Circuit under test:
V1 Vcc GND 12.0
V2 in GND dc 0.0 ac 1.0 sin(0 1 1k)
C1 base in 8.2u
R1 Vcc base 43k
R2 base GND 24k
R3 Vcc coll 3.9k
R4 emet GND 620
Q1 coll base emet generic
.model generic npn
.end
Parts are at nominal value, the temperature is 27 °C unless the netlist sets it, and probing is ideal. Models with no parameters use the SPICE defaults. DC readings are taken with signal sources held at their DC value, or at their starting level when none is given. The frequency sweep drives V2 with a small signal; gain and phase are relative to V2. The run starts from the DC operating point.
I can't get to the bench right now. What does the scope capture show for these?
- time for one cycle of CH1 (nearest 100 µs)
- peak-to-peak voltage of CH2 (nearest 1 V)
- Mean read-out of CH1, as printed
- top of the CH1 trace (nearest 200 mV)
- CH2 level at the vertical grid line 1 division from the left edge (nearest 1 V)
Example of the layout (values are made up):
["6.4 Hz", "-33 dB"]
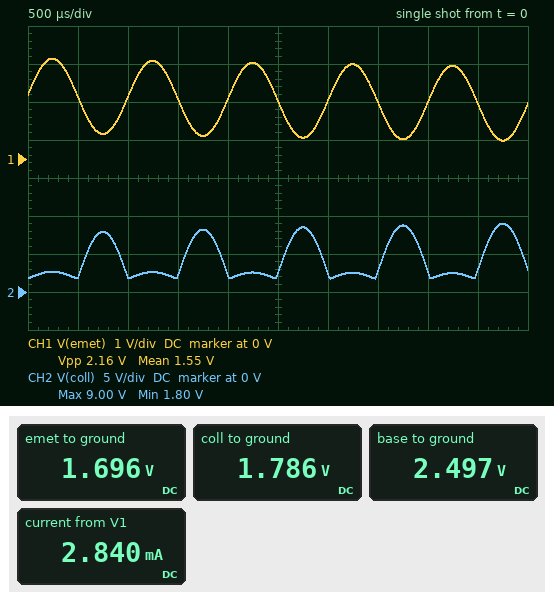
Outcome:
["1.0 ms", "7 V", "1.55 V", "2.6 V", "2 V"]
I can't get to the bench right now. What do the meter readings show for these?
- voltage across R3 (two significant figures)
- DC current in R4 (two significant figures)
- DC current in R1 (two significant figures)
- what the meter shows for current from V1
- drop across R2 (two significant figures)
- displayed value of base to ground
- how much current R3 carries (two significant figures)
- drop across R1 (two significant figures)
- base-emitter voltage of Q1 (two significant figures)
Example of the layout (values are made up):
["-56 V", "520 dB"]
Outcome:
["10 V", "2.7 mA", "220 µA", "2.840 mA", "2.5 V", "2.497 V", "2.6 mA", "9.5 V", "800 mV"]
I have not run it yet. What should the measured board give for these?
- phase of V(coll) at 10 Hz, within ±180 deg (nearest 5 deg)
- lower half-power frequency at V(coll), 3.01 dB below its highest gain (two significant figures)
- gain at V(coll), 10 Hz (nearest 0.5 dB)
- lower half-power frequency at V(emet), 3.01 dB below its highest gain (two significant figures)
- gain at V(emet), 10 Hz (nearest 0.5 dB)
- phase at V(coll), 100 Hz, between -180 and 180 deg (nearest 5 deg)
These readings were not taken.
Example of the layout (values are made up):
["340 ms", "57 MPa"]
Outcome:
["75 deg", "34 Hz", "-17.0 dB", "34 Hz", "-11.5 dB", "20 deg"]
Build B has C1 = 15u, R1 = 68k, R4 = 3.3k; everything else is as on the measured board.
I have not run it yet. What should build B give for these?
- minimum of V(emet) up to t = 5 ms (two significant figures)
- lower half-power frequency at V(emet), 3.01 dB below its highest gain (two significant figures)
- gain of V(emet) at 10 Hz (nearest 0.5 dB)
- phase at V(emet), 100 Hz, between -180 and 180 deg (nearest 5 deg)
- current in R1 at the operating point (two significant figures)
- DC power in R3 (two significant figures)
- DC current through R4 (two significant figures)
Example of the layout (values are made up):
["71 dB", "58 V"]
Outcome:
["1.3 V", "630 mHz", "0 dB", "0 deg", "130 µA", "1.8 mW", "680 µA"]
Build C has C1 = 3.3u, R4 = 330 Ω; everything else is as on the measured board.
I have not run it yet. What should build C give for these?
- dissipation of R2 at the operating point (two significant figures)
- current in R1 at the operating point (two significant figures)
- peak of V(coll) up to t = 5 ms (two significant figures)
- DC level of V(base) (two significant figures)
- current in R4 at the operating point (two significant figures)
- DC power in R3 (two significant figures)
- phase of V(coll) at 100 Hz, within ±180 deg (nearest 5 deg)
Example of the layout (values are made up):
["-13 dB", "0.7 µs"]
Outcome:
["130 µW", "240 µA", "12 V", "1.8 V", "3.0 mA", "31 mW", "55 deg"]
